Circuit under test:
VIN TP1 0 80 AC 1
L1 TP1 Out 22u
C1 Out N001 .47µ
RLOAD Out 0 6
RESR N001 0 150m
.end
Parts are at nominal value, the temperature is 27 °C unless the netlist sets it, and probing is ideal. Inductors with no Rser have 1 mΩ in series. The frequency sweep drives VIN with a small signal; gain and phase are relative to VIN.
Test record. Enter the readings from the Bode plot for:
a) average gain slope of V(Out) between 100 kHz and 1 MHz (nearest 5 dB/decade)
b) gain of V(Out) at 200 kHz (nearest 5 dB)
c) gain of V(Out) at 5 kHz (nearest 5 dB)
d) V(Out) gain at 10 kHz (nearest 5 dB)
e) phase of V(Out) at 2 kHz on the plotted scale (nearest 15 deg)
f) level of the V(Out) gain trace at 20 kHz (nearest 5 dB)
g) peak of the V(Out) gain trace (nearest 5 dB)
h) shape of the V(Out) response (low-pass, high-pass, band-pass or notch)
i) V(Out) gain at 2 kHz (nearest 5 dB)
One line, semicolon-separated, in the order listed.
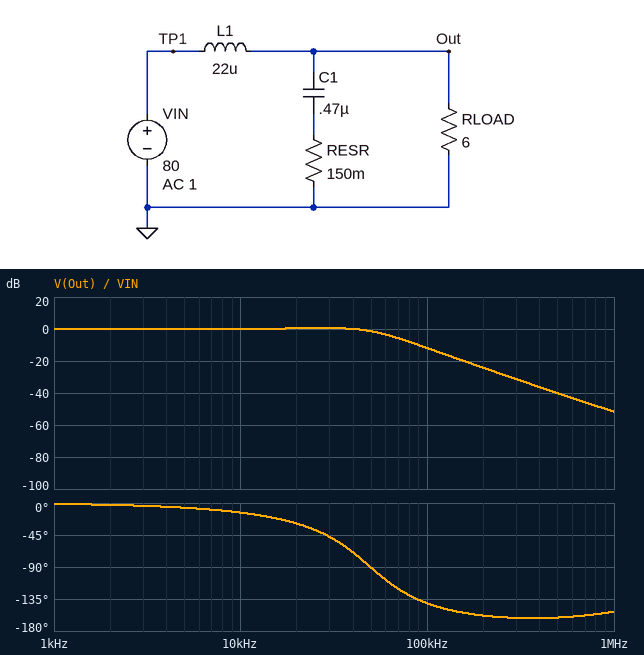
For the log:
-40 dB/decade; -25 dB; 0 dB; 0 dB; 0 deg; 0 dB; 0 dB; low-pass; 0 dB
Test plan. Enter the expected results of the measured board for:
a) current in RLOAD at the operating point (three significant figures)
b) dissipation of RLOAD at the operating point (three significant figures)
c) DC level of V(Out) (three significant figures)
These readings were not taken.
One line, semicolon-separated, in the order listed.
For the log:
13.3 A; 1.07 kW; 80.0 V
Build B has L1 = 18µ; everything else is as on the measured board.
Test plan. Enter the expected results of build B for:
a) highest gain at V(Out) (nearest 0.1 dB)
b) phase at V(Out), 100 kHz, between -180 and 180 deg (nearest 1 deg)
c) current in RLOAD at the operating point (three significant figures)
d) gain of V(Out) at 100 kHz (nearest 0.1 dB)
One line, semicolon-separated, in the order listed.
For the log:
1.0 dB; -139 deg; 13.3 A; -9.8 dB
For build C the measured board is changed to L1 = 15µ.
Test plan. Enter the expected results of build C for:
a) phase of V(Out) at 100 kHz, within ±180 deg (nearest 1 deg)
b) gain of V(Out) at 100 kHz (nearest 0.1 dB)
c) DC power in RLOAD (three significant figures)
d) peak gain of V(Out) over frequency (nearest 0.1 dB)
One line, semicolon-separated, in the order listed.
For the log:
-136 deg; -7.8 dB; 1.07 kW; 1.5 dB
